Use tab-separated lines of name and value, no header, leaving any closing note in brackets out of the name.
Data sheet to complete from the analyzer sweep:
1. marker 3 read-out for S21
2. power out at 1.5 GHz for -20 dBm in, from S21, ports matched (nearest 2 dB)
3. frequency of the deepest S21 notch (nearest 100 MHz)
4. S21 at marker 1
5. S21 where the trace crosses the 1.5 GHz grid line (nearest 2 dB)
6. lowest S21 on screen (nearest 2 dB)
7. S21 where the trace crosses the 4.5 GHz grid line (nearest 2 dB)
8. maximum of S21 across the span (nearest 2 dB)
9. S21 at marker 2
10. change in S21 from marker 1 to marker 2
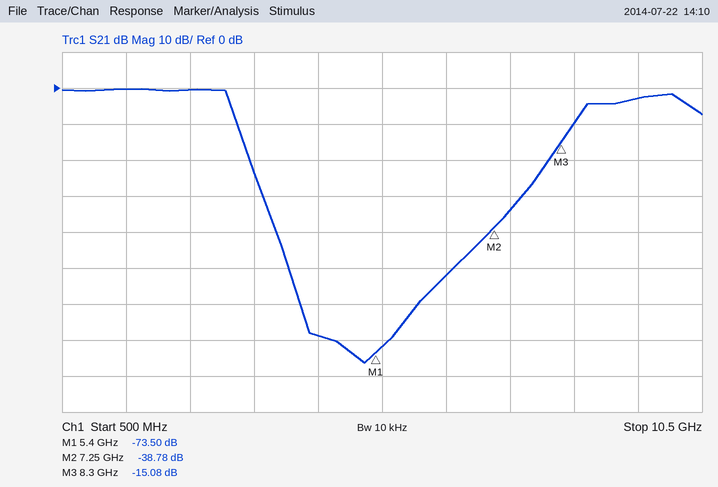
marker 3 read-out for S21	-15.08 dB
power out at 1.5 GHz for -20 dBm in, from S21, ports matched	-20 dBm
frequency of the deepest S21 notch	5.2 GHz
S21 at marker 1	-73.50 dB
S21 where the trace crosses the 1.5 GHz grid line	0 dB
lowest S21 on screen	-76 dB
S21 where the trace crosses the 4.5 GHz grid line	-68 dB
maximum of S21 across the span	0 dB
S21 at marker 2	-38.78 dB
change in S21 from marker 1 to marker 2	34.72 dB
